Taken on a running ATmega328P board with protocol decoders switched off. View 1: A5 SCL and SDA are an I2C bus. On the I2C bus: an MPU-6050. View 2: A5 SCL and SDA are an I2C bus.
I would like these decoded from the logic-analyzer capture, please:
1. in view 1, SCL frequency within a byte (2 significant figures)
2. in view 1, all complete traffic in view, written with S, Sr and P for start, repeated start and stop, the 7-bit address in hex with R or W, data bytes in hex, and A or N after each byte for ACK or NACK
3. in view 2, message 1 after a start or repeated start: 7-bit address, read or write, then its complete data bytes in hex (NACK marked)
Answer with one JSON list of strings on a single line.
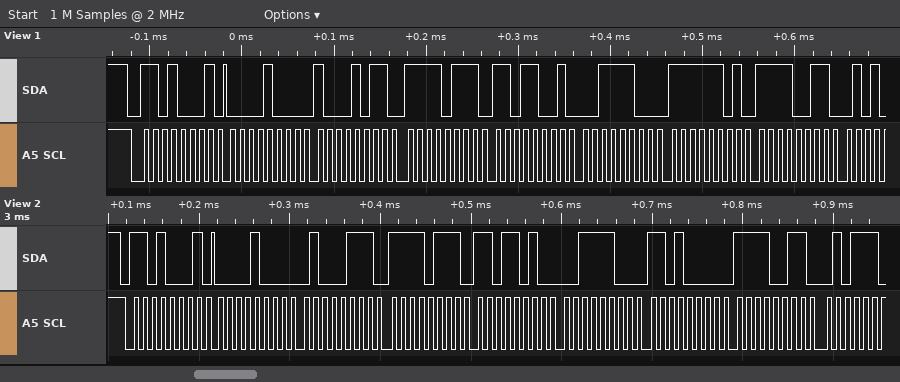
["100 kHz", "S 68R A 08 A 8B A F7 A D9 A 3C A FD A F3 A", "0x68 read: 08 47 F7 DA 3C D0 F3"]
